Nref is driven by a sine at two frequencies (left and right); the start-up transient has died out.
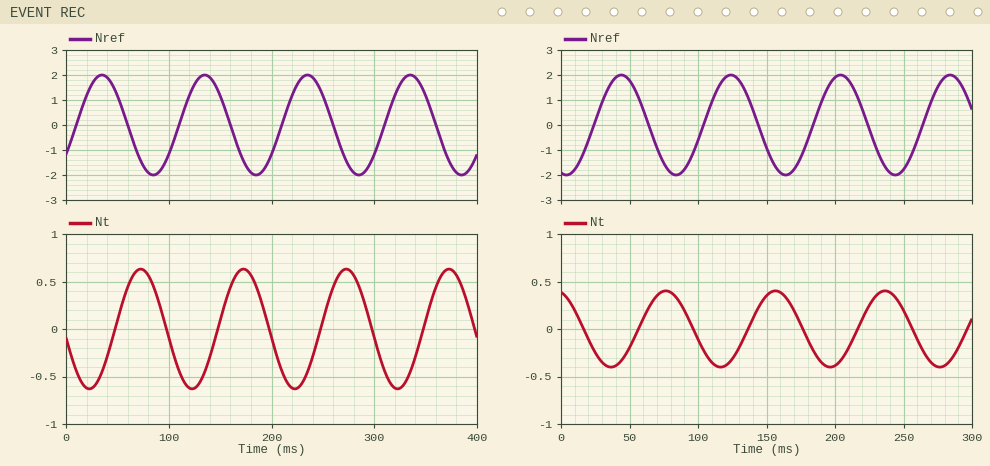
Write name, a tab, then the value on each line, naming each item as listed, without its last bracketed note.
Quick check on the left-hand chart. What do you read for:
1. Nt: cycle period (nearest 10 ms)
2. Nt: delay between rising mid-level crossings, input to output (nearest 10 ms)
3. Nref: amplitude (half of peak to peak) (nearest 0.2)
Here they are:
Nt: cycle period	100 ms
Nt: delay between rising mid-level crossings, input to output	40 ms
Nref: amplitude (half of peak to peak)	2.0
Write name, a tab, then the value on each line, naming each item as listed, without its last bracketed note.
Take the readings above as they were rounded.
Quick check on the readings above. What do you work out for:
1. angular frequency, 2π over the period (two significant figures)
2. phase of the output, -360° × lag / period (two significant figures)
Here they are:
angular frequency, 2π over the period	0.063 rad/ms
phase of the output, -360° × lag / period	-140°
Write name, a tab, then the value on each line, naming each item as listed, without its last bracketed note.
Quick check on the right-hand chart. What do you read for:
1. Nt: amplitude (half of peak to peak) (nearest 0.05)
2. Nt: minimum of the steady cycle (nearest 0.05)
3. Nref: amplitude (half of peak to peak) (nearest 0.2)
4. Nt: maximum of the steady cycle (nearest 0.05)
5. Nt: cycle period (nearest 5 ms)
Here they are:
Nt: amplitude (half of peak to peak)	0.40
Nt: minimum of the steady cycle	-0.40
Nref: amplitude (half of peak to peak)	2.0
Nt: maximum of the steady cycle	0.40
Nt: cycle period	80 ms
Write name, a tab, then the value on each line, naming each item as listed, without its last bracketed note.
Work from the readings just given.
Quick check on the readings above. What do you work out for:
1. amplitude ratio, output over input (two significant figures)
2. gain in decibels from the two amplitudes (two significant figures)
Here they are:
amplitude ratio, output over input	0.20
gain in decibels from the two amplitudes	-14 dB
